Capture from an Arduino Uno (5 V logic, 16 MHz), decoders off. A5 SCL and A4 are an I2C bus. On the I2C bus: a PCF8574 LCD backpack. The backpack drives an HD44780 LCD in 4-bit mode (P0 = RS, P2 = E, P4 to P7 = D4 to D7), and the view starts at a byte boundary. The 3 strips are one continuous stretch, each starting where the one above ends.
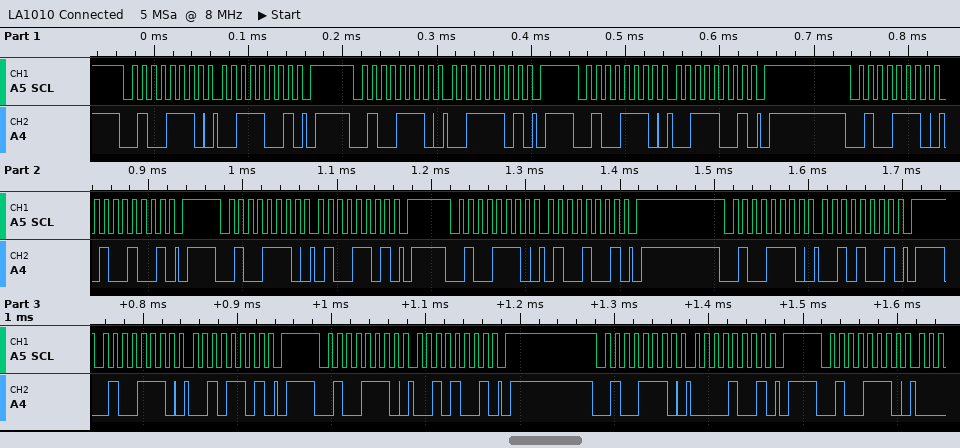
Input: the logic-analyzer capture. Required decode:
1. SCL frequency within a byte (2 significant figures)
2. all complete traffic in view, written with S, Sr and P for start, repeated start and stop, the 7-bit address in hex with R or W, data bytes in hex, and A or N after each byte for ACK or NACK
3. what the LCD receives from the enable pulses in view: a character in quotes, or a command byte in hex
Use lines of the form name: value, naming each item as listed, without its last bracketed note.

SCL frequency within a byte: 100 kHz
all complete traffic in view, written with S, Sr and P for start, repeated start and stop, the 7-bit address in hex with R or W, data bytes in hex, and A or N after each byte for ACK or NACK: S 27W A 39 A P S 27W A 3D A P S 27W A 39 A P S 27W A 49 A P S 27W A 4D A P S 27W A 49 A P S 27W A 29 A P S 27W A 2D A P S 27W A 29 A P S 27W A 09 A P S 27W A
what the LCD receives from the enable pulses in view: a character in quotes, or a command byte in hex: '4'
